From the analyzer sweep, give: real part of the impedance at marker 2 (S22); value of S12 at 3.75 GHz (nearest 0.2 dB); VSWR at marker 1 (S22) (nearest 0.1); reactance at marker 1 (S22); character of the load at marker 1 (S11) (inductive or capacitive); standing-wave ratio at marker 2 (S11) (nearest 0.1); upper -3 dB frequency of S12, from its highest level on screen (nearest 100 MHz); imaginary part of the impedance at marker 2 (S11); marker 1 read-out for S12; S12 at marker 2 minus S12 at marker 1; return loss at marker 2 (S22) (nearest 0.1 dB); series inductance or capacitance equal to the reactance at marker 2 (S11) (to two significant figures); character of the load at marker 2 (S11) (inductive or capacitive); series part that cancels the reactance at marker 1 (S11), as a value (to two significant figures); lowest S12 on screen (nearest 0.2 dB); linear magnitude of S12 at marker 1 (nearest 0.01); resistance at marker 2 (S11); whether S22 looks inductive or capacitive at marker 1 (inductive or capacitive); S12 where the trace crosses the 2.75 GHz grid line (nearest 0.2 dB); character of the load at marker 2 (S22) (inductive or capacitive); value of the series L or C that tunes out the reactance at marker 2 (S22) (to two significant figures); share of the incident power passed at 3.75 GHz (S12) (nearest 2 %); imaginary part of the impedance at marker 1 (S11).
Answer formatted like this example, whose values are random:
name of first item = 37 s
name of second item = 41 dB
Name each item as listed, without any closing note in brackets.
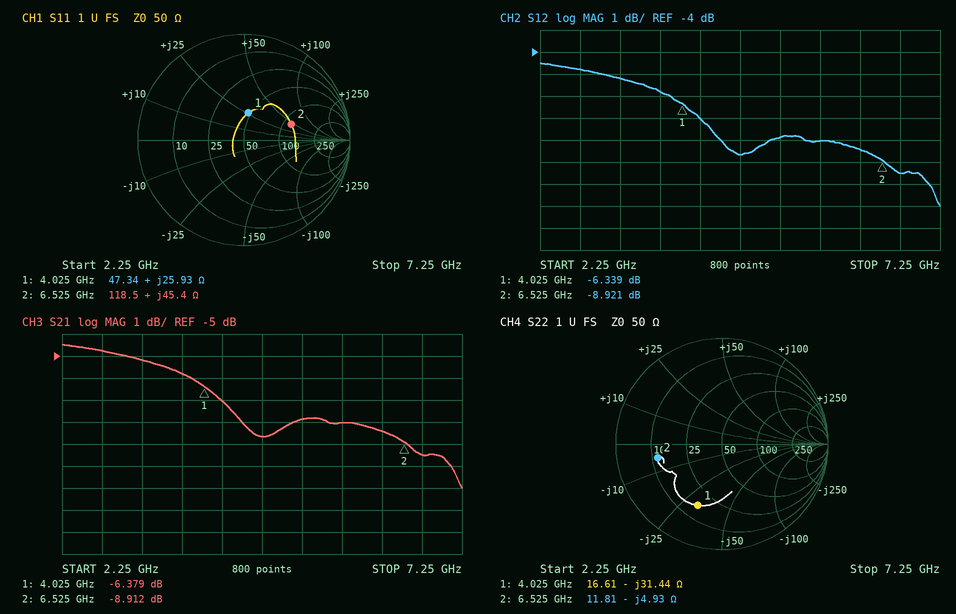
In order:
real part of the impedance at marker 2 = 11.81 Ω
value of S12 at 3.75 GHz = -5.8 dB
VSWR at marker 1 (S22) = 4.3
reactance at marker 1 = -31.44 Ω
character of the load at marker 1 (S11) = inductive
standing-wave ratio at marker 2 (S11) = 2.8
upper -3 dB frequency of S12, from its highest level on screen = 4.4 GHz
imaginary part of the impedance at marker 2 = +45.4 Ω
marker 1 read-out for S12 = -6.339 dB
S12 at marker 2 minus S12 at marker 1 = -2.582 dB
return loss at marker 2 (S22) = 4.1 dB
series inductance or capacitance equal to the reactance at marker 2 (S11) = 1.1 nH
character of the load at marker 2 (S11) = inductive
series part that cancels the reactance at marker 1 (S11), as a value = 1.5 pF
lowest S12 on screen = -11.0 dB
linear magnitude of S12 at marker 1 = 0.48
resistance at marker 2 = 118.5 Ω
whether S22 looks inductive or capacitive at marker 1 = capacitive
S12 where the trace crosses the 2.75 GHz grid line = -4.8 dB
character of the load at marker 2 (S22) = capacitive
value of the series L or C that tunes out the reactance at marker 2 (S22) = 120 pH
share of the incident power passed at 3.75 GHz (S12) = 26 %
imaginary part of the impedance at marker 1 = +25.93 Ω
